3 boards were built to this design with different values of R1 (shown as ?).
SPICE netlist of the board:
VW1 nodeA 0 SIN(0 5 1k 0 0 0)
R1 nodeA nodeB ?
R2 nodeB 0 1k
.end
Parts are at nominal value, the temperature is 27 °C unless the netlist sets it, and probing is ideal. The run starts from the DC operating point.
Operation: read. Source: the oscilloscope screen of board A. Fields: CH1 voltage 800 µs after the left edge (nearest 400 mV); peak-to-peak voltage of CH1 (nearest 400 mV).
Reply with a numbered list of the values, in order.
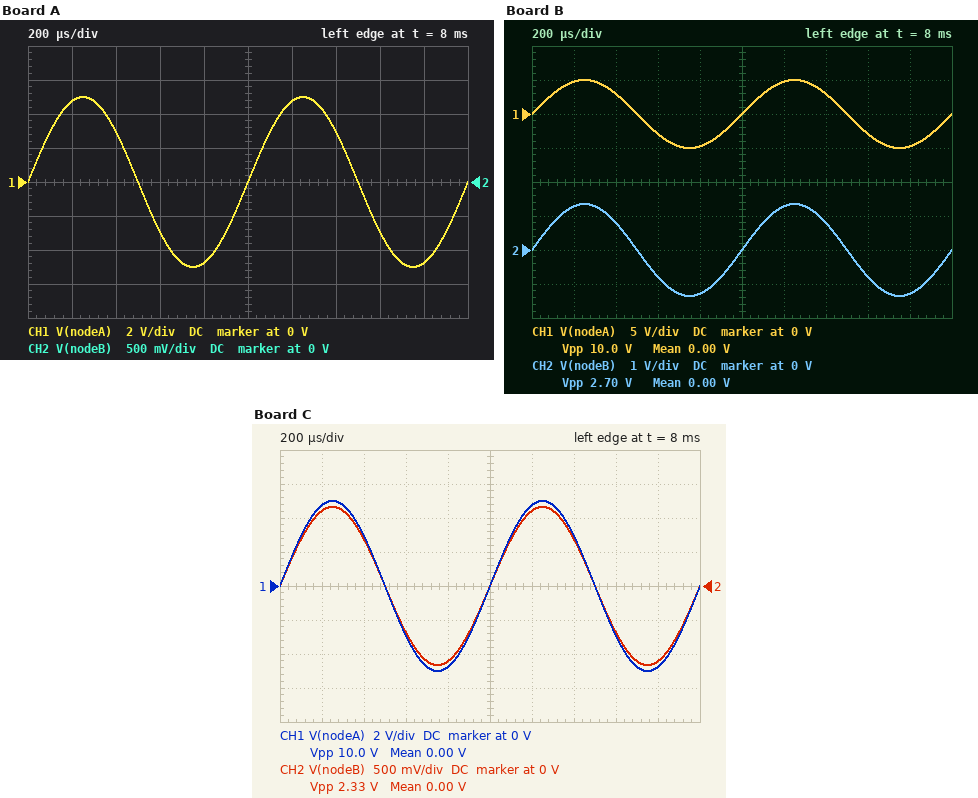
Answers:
1. -4.8 V
2. 10.0 V
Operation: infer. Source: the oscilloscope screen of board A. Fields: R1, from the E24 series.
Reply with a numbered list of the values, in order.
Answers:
1. 3 kΩ
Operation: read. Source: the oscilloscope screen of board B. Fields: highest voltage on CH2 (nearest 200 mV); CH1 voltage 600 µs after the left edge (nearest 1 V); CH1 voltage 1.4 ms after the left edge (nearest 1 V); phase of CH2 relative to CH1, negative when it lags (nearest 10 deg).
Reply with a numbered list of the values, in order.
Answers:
1. 1.4 V
2. -3 V
3. 3 V
4. 0 deg
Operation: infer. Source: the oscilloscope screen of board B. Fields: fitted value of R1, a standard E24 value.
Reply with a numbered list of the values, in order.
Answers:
1. 2.7 kΩ
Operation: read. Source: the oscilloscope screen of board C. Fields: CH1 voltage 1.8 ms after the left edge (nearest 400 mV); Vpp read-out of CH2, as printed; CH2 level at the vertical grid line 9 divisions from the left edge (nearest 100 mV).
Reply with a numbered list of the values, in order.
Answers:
1. -4.8 V
2. 2.33 V
3. -1.1 V
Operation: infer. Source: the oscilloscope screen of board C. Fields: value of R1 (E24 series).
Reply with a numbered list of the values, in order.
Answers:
1. 3.3 kΩ
